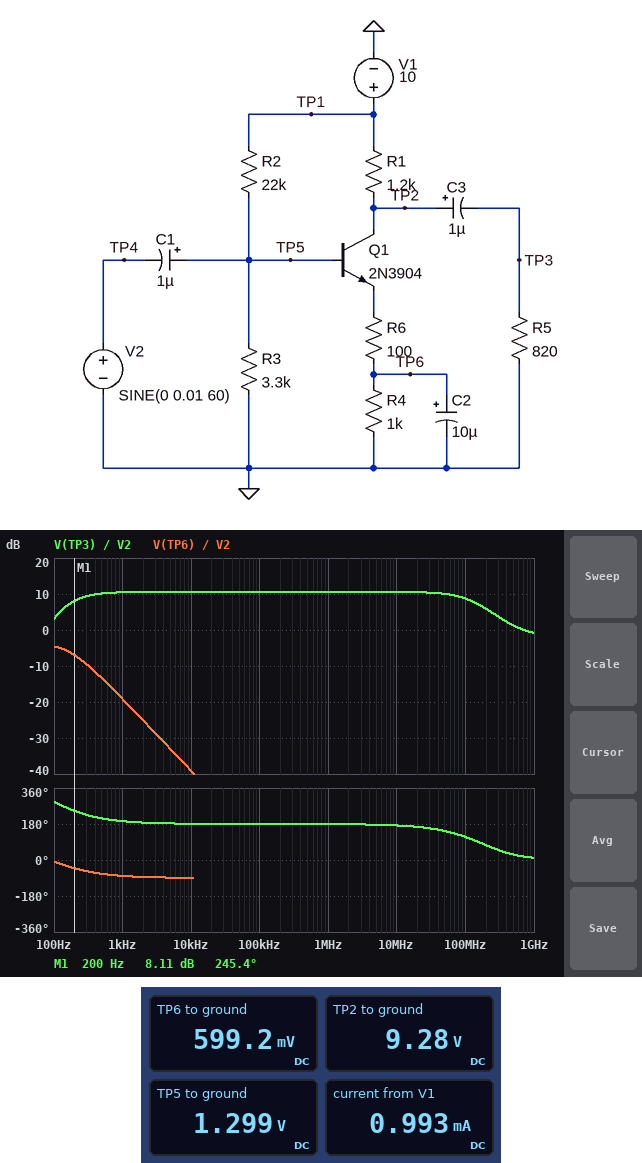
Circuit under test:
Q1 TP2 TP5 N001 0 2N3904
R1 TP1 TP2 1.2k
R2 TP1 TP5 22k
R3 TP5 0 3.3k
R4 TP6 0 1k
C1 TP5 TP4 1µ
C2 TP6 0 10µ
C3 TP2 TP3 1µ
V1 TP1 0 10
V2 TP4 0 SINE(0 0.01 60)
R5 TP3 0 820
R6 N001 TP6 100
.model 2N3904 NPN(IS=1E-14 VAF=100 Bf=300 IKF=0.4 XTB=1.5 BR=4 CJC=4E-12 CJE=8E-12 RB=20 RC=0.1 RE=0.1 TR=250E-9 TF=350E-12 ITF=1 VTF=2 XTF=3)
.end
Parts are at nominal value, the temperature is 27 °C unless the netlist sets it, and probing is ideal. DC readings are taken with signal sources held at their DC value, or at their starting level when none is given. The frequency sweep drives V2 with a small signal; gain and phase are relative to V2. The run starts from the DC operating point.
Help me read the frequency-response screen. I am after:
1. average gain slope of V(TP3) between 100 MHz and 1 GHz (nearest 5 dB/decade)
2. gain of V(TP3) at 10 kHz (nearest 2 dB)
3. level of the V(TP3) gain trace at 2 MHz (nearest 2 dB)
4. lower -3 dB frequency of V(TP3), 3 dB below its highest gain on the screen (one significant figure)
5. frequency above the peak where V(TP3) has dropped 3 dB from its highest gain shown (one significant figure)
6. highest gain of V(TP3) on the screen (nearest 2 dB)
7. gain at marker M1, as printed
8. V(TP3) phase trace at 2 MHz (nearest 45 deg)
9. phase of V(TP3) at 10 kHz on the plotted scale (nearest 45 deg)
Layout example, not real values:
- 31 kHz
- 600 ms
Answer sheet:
- -10 dB/decade
- 10 dB
- 10 dB
- 200 Hz
- 100 MHz
- 10 dB
- 8.11 dB
- 180 deg
- 180 deg
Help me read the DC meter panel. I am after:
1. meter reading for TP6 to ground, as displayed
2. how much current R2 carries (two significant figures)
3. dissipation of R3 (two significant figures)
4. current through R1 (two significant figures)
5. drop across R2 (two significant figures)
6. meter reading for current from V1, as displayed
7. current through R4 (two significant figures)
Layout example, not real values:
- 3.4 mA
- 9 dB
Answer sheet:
- 599.2 mV
- 400 µA
- 510 µW
- 600 µA
- 8.7 V
- 0.993 mA
- 600 µA
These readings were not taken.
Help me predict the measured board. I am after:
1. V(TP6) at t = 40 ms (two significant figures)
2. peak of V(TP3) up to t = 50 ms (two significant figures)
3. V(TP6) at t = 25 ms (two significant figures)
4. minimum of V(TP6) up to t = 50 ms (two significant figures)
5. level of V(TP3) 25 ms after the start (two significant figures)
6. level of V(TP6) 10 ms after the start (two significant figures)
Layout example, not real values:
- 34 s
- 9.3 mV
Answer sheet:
- 600 mV
- 6.5 mV
- 600 mV
- 590 mV
- 3.7 mV
- 590 mV
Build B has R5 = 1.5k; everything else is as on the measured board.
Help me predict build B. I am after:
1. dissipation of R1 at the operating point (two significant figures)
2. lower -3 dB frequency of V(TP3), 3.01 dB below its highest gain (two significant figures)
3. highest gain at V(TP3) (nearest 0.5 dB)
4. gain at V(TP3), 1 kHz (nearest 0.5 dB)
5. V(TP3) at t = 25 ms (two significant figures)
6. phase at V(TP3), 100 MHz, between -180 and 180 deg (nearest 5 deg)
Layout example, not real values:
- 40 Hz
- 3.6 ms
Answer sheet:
- 430 µW
- 170 Hz
- 13.5 dB
- 13.0 dB
- 7.2 mV
- 105 deg
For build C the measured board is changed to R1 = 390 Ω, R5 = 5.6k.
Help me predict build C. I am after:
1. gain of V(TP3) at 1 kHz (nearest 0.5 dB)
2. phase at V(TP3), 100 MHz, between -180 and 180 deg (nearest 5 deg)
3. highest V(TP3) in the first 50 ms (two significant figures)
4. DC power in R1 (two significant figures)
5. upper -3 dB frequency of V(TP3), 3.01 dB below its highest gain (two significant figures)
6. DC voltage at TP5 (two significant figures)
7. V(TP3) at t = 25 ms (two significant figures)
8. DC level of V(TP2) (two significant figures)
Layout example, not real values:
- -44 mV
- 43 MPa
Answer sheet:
- 8.0 dB
- 120 deg
- 7.4 mV
- 140 µW
- 180 MHz
- 1.3 V
- 6.6 mV
- 9.8 V
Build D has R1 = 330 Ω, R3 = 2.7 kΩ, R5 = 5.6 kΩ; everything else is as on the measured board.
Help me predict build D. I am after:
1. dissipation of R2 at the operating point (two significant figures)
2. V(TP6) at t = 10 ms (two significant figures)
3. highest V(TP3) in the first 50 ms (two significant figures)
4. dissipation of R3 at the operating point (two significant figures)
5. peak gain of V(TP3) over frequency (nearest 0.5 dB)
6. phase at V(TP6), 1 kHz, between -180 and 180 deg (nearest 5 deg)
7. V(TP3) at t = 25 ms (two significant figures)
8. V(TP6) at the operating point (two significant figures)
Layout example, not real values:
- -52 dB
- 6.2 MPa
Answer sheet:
- 3.6 mW
- 410 mV
- 5.6 mV
- 440 µW
- 5.5 dB
- -80 deg
- 4.9 mV
- 420 mV
